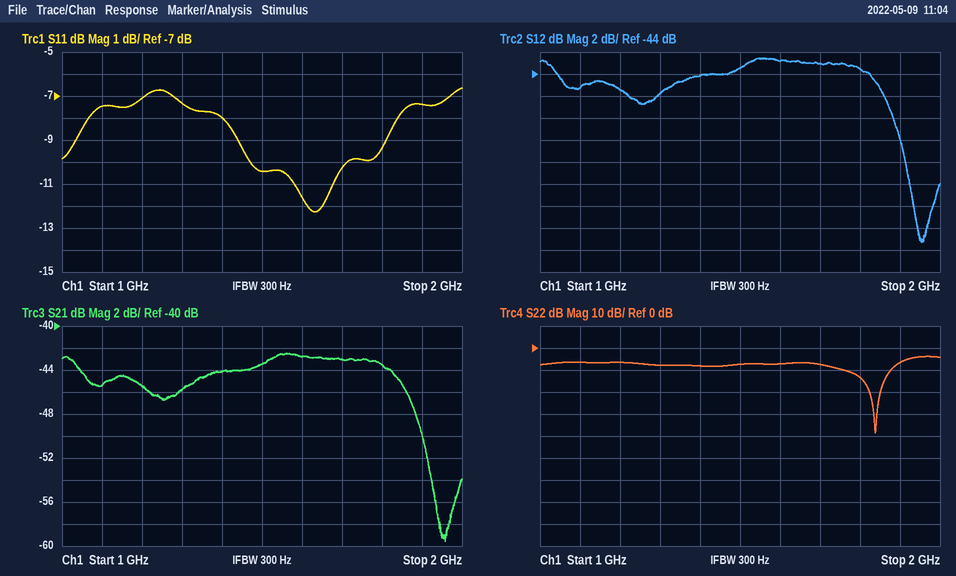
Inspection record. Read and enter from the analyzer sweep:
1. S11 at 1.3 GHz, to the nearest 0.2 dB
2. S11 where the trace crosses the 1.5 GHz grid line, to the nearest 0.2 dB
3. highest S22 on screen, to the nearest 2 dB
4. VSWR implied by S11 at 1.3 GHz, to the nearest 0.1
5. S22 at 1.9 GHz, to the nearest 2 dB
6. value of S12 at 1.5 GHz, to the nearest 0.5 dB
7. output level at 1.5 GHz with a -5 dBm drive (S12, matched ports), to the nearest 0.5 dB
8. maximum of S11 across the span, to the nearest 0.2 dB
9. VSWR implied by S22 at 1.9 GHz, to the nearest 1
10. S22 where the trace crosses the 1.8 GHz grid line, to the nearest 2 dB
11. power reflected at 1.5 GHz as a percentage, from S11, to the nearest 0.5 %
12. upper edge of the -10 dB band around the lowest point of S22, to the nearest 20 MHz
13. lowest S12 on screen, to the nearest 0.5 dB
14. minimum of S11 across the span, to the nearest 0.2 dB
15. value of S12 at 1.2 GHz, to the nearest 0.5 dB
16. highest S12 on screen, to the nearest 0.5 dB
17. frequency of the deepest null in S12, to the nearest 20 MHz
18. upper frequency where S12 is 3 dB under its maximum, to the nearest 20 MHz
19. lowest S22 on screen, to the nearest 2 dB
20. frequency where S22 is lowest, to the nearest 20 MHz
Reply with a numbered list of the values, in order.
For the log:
1. -7.4 dB
2. -10.4 dB
3. -4 dB
4. 2.5
5. -6 dB
6. -43.5 dB
7. -48.5 dBm
8. -6.6 dB
9. 3
10. -14 dB
11. 9.0 %
12. 1.88 GHz
13. -59.5 dB
14. -12.2 dB
15. -45.5 dB
16. -42.5 dB
17. 1.96 GHz
18. 1.86 GHz
19. -38 dB
20. 1.84 GHz
